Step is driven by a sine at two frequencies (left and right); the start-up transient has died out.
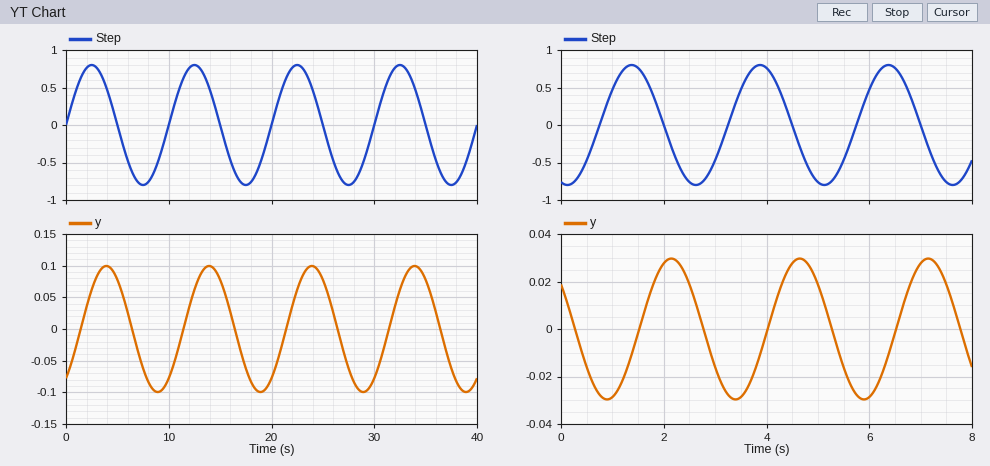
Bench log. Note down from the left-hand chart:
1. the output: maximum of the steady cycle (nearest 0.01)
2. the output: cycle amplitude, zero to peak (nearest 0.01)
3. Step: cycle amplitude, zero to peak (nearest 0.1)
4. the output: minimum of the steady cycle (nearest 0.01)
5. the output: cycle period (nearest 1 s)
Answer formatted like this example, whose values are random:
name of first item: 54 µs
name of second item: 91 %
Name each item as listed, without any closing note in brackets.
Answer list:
the output: maximum of the steady cycle: 0.10
the output: cycle amplitude, zero to peak: 0.10
Step: cycle amplitude, zero to peak: 0.8
the output: minimum of the steady cycle: -0.10
the output: cycle period: 10 s
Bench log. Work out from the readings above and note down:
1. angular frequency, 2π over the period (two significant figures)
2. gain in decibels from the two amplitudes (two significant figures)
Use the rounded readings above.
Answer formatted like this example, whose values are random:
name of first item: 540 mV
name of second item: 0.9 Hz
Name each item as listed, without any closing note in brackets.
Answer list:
angular frequency, 2π over the period: 0.63 rad/s
gain in decibels from the two amplitudes: -18 dB
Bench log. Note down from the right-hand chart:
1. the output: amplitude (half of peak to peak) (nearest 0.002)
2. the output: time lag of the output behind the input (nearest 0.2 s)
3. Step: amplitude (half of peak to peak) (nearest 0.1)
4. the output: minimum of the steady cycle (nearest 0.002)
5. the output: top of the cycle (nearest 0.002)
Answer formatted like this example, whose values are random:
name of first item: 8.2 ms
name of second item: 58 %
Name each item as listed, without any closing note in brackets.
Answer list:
the output: amplitude (half of peak to peak): 0.030
the output: time lag of the output behind the input: 0.8 s
Step: amplitude (half of peak to peak): 0.8
the output: minimum of the steady cycle: -0.030
the output: top of the cycle: 0.030
